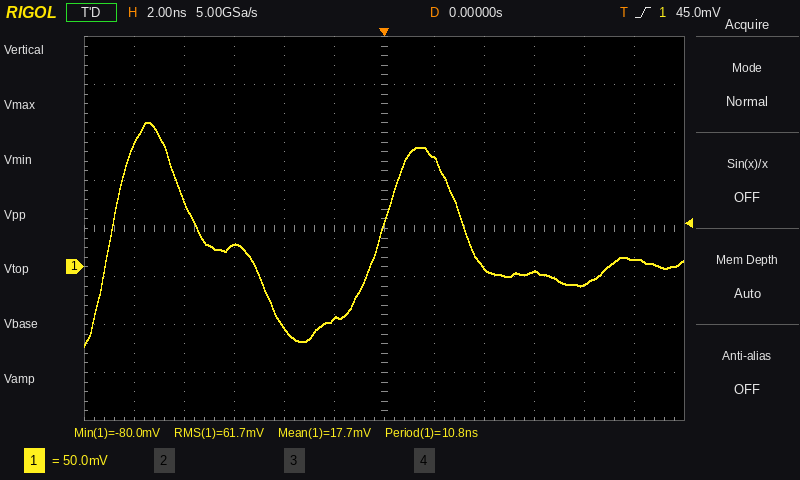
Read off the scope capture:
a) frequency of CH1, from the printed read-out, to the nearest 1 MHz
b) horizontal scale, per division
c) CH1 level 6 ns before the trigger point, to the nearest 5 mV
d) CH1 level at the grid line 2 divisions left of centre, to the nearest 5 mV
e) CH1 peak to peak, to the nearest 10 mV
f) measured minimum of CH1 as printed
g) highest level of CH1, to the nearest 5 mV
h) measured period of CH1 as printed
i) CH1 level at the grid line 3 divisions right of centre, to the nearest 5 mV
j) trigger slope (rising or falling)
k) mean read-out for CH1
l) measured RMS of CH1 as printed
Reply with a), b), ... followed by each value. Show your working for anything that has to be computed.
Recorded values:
a) 1 / 10.8 ns ≈ 93 MHz
b) 2 ns
c) 25 mV
d) -65 mV
e) 230 mV
f) -80.0 mV
g) 150 mV
h) 10.8 ns
i) -5 mV
j) rising
k) 17.7 mV
l) 61.7 mV
